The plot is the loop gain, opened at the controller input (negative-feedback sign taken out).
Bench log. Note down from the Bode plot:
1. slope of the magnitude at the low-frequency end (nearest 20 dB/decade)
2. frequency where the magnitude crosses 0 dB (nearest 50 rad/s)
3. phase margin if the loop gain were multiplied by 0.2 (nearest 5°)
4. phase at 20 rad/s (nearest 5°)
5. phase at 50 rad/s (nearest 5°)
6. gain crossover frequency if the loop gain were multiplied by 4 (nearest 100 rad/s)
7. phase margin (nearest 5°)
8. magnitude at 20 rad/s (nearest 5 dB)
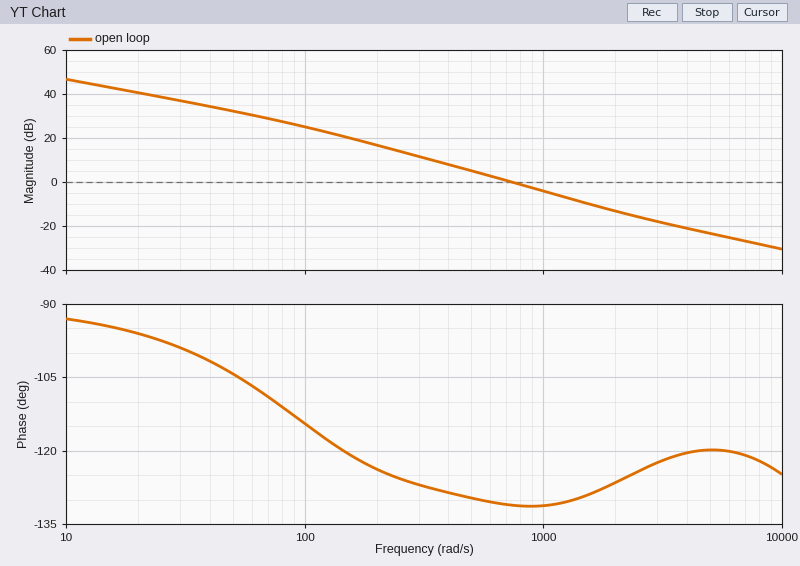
-20 dB/decade
750 rad/s
55°
-95°
-105°
1800 rad/s
50°
40 dB
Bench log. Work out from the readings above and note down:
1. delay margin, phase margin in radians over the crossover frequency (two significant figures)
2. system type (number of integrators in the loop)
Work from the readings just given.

0.0012 s
1
